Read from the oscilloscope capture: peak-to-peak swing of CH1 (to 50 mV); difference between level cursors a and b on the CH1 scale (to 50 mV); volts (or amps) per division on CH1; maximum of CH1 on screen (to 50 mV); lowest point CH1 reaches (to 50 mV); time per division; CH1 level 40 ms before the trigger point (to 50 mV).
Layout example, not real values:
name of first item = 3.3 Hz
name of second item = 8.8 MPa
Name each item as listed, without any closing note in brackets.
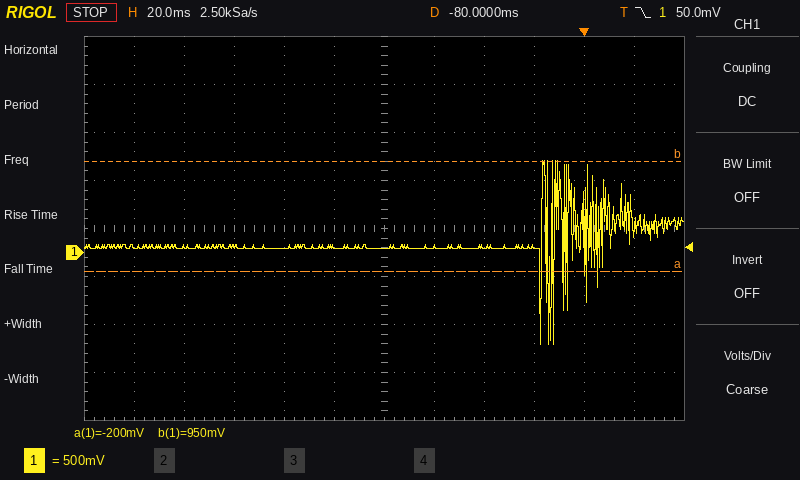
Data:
peak-to-peak swing of CH1 = 1.90 V
difference between level cursors a and b on the CH1 scale = 1.15 V
volts (or amps) per division on CH1 = 500 mV
maximum of CH1 on screen = 950 mV
lowest point CH1 reaches = -950 mV
time per division = 20 ms
CH1 level 40 ms before the trigger point = 50 mV
